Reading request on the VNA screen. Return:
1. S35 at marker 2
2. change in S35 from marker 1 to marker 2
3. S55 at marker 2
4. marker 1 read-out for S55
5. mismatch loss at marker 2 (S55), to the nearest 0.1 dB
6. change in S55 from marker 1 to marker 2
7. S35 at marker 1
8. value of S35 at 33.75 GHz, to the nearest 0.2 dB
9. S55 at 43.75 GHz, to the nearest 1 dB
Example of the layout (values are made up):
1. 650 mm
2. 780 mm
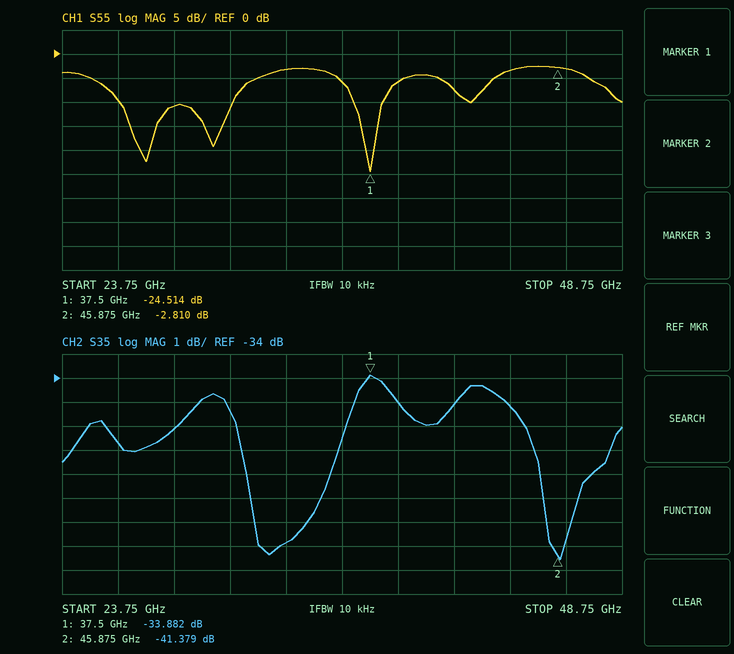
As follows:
1. -41.379 dB
2. -7.497 dB
3. -2.810 dB
4. -24.514 dB
5. 3.2 dB
6. 21.704 dB
7. -33.882 dB
8. -40.8 dB
9. -3 dB
